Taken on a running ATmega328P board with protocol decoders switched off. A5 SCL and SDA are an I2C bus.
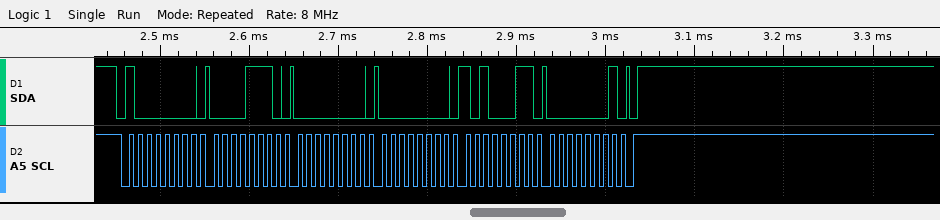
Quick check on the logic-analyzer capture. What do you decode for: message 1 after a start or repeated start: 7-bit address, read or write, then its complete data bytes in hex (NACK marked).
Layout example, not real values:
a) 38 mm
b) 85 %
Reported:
a) 0x40 write: 0E 00 00 A3 01
